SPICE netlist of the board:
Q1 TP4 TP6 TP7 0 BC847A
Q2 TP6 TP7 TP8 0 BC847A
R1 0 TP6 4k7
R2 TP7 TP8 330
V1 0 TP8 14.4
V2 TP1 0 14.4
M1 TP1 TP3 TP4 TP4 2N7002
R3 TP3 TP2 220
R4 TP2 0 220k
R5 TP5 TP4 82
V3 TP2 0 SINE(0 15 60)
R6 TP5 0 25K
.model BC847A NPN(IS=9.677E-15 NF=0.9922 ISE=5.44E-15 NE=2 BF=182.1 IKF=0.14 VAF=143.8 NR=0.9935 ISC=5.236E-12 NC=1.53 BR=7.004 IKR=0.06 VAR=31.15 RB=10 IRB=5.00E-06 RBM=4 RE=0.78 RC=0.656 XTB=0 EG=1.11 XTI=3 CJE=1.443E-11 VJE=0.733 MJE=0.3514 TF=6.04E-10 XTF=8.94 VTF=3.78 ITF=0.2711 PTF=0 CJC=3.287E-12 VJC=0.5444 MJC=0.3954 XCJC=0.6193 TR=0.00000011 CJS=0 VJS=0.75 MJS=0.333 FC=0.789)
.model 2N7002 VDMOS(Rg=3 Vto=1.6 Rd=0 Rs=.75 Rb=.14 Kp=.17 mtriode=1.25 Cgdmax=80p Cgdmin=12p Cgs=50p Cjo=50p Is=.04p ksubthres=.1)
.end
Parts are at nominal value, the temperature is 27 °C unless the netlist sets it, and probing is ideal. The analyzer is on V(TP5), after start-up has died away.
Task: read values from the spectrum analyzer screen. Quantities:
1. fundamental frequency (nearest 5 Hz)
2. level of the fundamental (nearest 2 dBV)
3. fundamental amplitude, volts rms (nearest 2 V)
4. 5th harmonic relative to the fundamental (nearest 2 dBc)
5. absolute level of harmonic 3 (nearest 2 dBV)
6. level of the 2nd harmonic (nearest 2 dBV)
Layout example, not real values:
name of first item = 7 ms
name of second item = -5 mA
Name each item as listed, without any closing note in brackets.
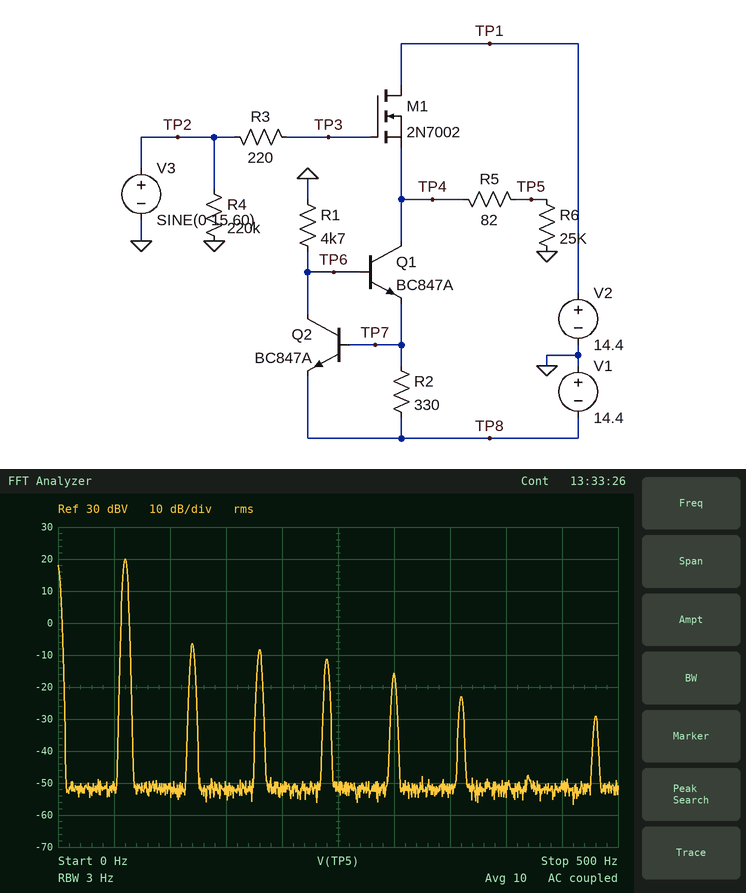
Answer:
fundamental frequency = 60 Hz
level of the fundamental = 20 dBV
fundamental amplitude, volts rms = 10 V
5th harmonic relative to the fundamental = -36 dBc
absolute level of harmonic 3 = -8 dBV
level of the 2nd harmonic = -6 dBV
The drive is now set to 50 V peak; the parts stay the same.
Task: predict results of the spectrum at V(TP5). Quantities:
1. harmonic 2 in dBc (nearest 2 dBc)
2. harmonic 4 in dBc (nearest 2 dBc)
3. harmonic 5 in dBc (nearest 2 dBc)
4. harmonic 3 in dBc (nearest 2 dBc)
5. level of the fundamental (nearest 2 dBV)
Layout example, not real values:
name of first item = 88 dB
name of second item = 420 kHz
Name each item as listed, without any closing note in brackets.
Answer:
harmonic 2 in dBc = -28 dBc
harmonic 4 in dBc = -30 dBc
harmonic 5 in dBc = -18 dBc
harmonic 3 in dBc = -10 dBc
level of the fundamental = 22 dBV
